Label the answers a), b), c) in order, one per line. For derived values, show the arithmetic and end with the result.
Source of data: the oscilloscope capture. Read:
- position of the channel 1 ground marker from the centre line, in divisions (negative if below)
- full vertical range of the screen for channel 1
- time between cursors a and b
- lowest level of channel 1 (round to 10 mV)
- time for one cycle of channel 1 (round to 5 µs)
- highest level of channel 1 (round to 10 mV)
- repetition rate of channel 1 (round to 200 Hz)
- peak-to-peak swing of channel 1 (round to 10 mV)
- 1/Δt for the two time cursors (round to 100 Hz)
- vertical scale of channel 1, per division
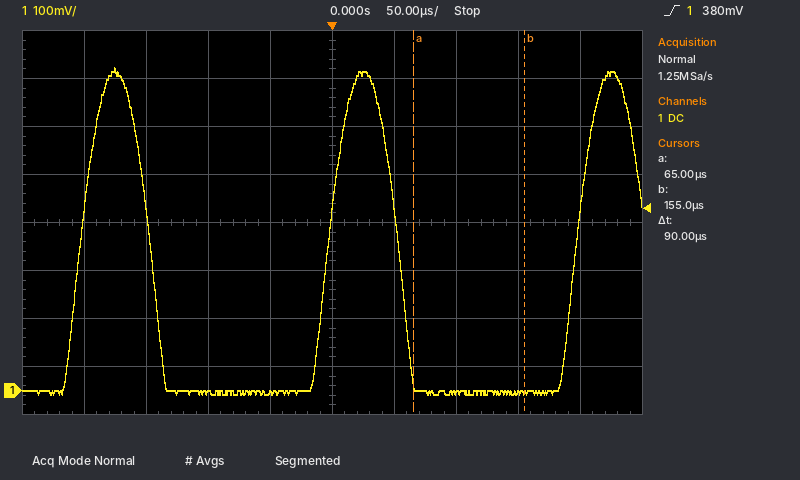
a) -3.5 div
b) 800 mV
c) 90 µs
d) -10 mV
e) 200 µs
f) 670 mV
g) 1 / 200 µs ≈ 5.0 kHz
h) 670 mV − (-10 mV) = 680 mV
i) 1 / 90 µs ≈ 11.1 kHz
j) 100 mV
